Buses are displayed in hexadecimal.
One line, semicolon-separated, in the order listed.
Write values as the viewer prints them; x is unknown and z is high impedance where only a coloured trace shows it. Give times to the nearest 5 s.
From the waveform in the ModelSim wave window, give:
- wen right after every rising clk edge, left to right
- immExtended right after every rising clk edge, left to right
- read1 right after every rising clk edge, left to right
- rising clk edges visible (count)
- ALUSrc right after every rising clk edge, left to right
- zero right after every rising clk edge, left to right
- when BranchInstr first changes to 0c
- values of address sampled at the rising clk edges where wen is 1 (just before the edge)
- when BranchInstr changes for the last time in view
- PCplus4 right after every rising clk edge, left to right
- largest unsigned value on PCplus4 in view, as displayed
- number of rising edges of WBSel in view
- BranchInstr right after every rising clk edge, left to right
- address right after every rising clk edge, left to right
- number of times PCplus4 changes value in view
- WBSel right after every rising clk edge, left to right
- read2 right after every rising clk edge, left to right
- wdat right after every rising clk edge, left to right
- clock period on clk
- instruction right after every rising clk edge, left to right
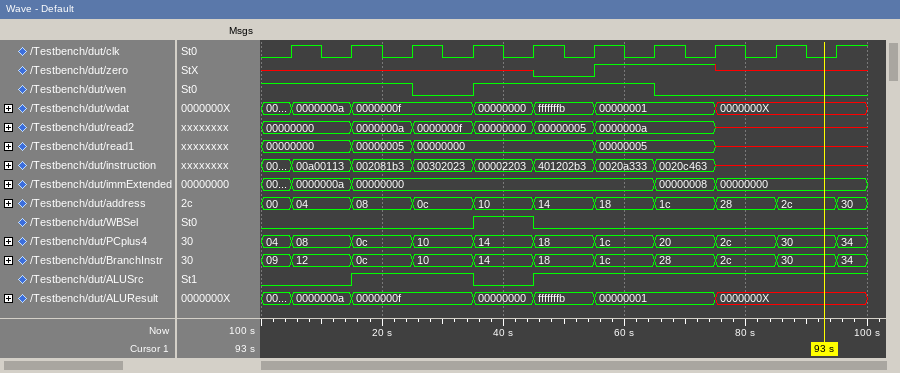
1 1 0 1 1 1 0 0 0 0; 0000000a, 00000000, 00000000, 00000000, 00000000, 00000000, 00000008, 00000000, 00000000, 00000000; 00000000, 00000005, 00000000, 00000000, 00000000, 00000005, 00000005, x, x, x; 10; 0 1 1 0 1 1 1 1 1 1; x x x x 0 1 1 x x x; 15 s; 00, 04, 08, 10, 14, 18; 95 s; 08, 0c, 10, 14, 18, 1c, 20, 2c, 30, 34; 34; 1; 12, 0c, 10, 14, 18, 1c, 28, 2c, 30, 34; 04, 08, 0c, 10, 14, 18, 1c, 28, 2c, 30; 10; 0 0 0 1 0 0 0 0 0 0; 00000000, 0000000a, 0000000f, 00000000, 00000005, 0000000a, 0000000a, x, x, x; 0000000a, 0000000f, 0000000f, 00000000, fffffffb, 00000001, 00000001, 0000000X, 0000000X, 0000000X; 10 s; 00a00113, 002081b3, 00302023, 00002203, 401202b3, 0020a333, 0020c463, x, x, x
